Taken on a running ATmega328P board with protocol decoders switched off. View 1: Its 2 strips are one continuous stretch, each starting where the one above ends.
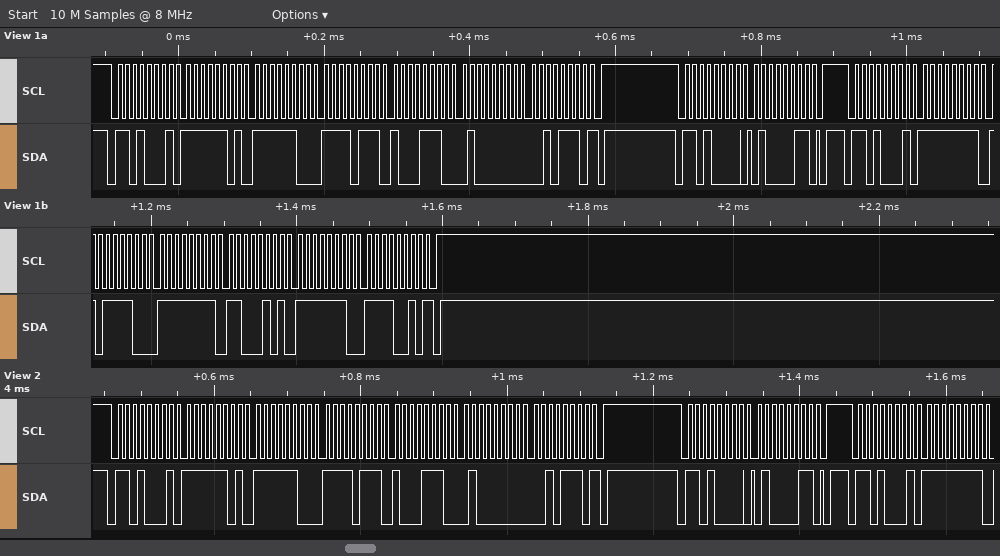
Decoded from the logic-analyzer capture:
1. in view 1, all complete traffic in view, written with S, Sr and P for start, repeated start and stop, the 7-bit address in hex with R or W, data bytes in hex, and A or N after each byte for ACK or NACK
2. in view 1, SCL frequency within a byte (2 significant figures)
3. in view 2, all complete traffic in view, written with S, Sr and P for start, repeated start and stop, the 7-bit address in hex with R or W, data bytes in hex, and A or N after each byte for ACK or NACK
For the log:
S 68R A FD A FC A F7 A 8E A 40 A 2E N P S 68W A 43 A P S 68R A FF A BC A FF A C5 A FE A F2 N P
100 kHz
S 68R A FD A FC A F7 A 8E A 40 A 2E N P S 68W A 43 A P S 68R A FF A
